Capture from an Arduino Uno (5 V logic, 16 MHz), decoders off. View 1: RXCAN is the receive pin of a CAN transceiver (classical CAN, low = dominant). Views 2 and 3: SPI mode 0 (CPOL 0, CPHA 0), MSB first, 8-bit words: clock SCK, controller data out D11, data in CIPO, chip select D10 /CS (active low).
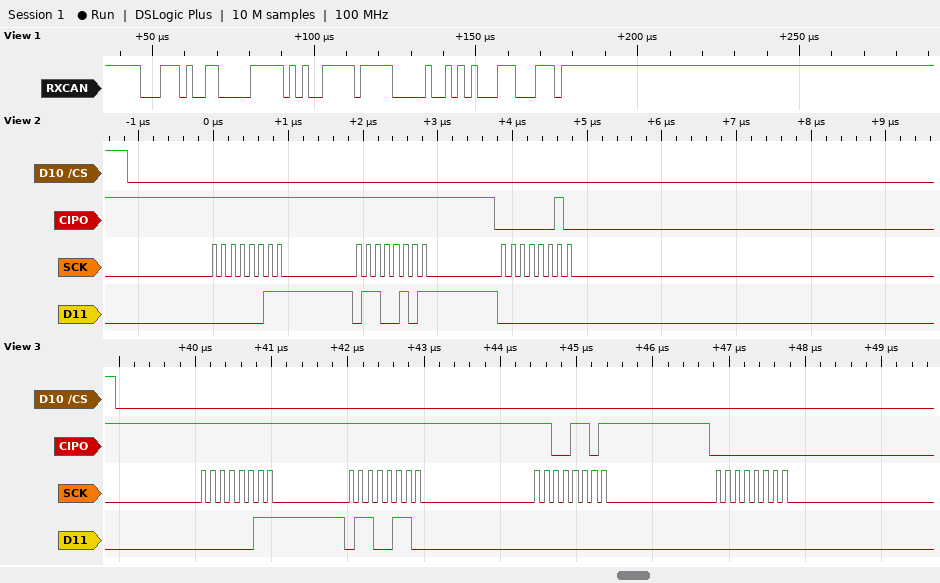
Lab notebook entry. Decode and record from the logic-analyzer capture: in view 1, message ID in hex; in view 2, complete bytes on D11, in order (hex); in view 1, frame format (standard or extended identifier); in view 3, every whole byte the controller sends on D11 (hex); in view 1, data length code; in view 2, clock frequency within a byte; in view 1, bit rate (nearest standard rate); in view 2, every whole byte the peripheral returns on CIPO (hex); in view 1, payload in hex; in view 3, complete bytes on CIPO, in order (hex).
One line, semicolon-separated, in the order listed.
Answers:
0x1D3; 0x03 0x65 0x00; standard; 0x03 0x66 0x00 0x00; 3; 8 MHz; 500 kbit/s; 0xFF 0xFF 0x02; E9 FF 81; 0xFF 0xFF 0xCD 0x00
